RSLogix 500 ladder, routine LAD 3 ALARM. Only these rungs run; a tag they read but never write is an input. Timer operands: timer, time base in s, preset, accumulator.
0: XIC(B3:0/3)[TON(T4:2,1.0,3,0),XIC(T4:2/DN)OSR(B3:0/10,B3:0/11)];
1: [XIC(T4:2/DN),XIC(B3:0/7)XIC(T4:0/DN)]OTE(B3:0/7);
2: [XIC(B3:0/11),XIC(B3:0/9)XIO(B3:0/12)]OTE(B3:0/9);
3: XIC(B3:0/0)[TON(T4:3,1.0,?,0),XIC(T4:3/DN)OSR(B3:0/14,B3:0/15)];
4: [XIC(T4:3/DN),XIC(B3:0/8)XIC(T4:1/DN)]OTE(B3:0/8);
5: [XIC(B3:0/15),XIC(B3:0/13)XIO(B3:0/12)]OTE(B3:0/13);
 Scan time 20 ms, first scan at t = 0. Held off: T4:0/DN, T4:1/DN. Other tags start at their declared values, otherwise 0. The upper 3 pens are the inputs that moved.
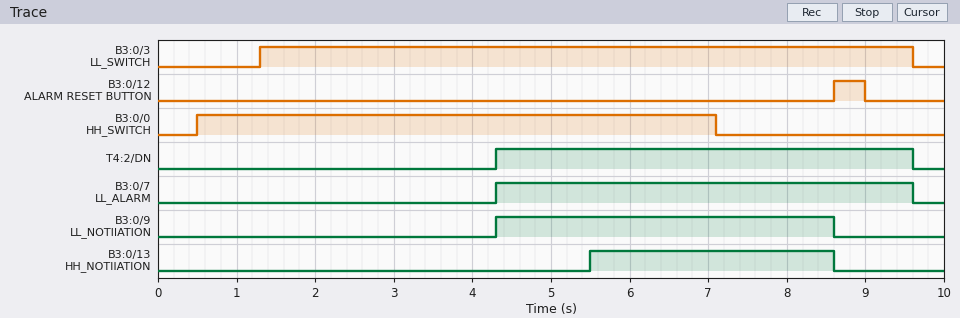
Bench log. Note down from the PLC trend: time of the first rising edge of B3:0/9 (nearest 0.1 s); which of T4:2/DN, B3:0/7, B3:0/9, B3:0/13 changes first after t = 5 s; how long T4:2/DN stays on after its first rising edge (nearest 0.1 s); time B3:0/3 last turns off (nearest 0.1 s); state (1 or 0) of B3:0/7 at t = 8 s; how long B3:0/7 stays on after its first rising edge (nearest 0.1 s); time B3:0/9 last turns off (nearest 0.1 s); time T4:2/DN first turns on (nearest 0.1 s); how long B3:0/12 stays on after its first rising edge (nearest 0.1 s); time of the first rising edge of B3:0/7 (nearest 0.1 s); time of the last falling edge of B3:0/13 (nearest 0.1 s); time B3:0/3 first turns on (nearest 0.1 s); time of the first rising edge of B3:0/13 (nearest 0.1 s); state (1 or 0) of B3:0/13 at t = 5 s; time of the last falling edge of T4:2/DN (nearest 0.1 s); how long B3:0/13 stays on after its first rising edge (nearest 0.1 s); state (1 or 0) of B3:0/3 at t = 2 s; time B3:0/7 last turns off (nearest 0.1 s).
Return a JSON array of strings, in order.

["4.3 s", "B3:0/13", "5.3 s", "9.6 s", "1", "5.3 s", "8.6 s", "4.3 s", "0.4 s", "4.3 s", "8.6 s", "1.3 s", "5.5 s", "0", "9.6 s", "3.1 s", "1", "9.6 s"]
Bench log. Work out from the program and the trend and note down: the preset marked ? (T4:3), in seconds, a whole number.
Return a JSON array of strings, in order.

["5 s"]
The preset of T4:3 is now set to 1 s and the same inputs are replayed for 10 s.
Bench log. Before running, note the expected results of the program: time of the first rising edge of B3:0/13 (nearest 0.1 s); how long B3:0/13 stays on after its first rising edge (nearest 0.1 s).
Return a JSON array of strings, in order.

["1.5 s", "7.1 s"]
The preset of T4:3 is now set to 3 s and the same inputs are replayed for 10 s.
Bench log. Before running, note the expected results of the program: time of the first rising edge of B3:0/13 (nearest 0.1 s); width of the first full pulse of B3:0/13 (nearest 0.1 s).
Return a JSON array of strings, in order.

["3.5 s", "5.1 s"]
